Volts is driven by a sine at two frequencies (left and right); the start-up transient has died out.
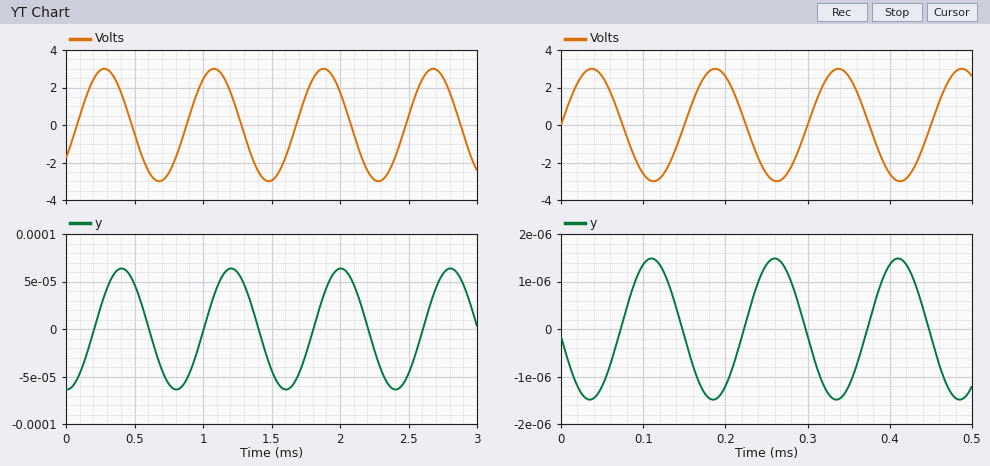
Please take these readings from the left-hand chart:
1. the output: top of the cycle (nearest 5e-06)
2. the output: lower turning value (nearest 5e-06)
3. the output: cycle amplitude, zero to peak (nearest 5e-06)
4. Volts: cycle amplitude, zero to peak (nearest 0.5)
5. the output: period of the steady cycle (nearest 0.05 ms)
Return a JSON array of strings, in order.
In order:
["0.000065", "-0.000065", "0.000065", "3.0", "0.80 ms"]
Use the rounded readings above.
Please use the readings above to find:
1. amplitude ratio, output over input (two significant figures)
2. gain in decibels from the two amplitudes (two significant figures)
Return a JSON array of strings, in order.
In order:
["0.000022", "-93 dB"]
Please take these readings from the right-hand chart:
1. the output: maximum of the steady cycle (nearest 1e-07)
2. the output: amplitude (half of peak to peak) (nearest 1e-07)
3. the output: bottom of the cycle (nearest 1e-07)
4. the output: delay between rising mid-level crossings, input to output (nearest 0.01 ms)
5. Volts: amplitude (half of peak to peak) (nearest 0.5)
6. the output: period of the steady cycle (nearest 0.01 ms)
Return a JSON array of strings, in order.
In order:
["0.0000015", "0.0000015", "-0.0000015", "0.07 ms", "3.0", "0.15 ms"]
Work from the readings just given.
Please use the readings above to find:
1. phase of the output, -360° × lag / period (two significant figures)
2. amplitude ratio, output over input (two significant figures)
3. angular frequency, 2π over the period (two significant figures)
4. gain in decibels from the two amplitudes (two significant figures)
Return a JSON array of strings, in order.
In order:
["-170°", "0.00000050", "42 rad/ms", "-130 dB"]
